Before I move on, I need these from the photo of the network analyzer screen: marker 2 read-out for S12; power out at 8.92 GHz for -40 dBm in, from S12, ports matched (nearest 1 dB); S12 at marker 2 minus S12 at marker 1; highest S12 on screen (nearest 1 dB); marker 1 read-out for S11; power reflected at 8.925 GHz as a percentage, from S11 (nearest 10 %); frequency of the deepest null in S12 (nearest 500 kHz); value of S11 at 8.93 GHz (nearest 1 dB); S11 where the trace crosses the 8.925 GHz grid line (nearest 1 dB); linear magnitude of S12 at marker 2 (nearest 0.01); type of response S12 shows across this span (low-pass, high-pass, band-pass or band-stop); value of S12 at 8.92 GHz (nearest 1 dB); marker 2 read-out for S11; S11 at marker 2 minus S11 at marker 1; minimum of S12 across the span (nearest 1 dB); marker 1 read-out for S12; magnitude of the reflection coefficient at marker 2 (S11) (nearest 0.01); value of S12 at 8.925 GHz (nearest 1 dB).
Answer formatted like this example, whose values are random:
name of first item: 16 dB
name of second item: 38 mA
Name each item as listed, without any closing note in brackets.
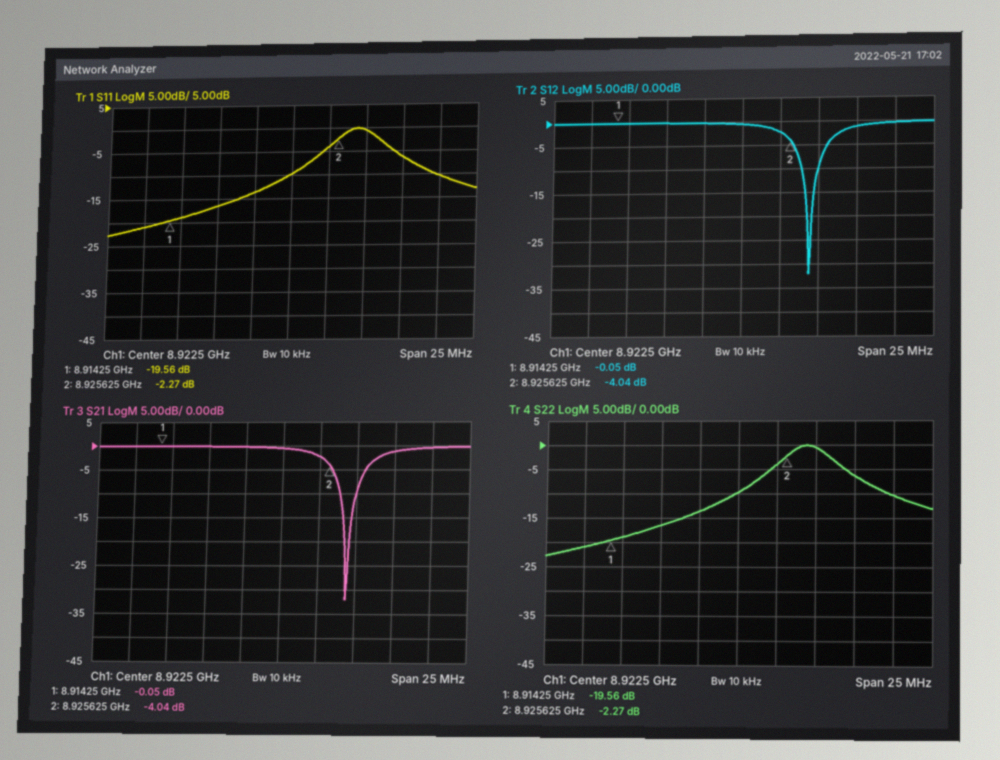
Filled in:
marker 2 read-out for S12: -4.04 dB
power out at 8.92 GHz for -40 dBm in, from S12, ports matched: -40 dBm
S12 at marker 2 minus S12 at marker 1: -3.99 dB
highest S12 on screen: 0 dB
marker 1 read-out for S11: -19.56 dB
power reflected at 8.925 GHz as a percentage, from S11: 40 %
frequency of the deepest null in S12: 8.9270 GHz
value of S11 at 8.93 GHz: -6 dB
S11 where the trace crosses the 8.925 GHz grid line: -4 dB
linear magnitude of S12 at marker 2: 0.63
type of response S12 shows across this span: band-stop
value of S12 at 8.92 GHz: 0 dB
marker 2 read-out for S11: -2.27 dB
S11 at marker 2 minus S11 at marker 1: 17.29 dB
minimum of S12 across the span: -32 dB
marker 1 read-out for S12: -0.05 dB
magnitude of the reflection coefficient at marker 2 (S11): 0.77
value of S12 at 8.925 GHz: -2 dB
